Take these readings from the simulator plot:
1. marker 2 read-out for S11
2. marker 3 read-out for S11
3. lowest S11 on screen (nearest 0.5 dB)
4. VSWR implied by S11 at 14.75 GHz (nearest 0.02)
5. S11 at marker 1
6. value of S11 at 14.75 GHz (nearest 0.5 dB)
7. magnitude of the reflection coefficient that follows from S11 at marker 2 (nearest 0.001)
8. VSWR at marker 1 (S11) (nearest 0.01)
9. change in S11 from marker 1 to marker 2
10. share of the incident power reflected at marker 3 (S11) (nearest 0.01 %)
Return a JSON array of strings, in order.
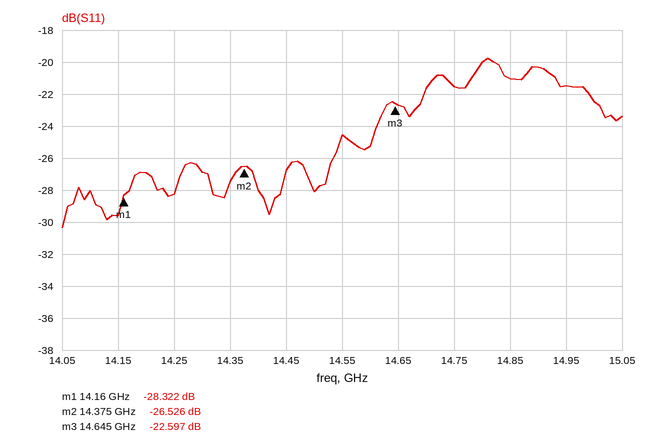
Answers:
["-26.526 dB", "-22.597 dB", "-30.5 dB", "1.18", "-28.322 dB", "-21.5 dB", "0.047", "1.08", "1.796 dB", "0.55 %"]
